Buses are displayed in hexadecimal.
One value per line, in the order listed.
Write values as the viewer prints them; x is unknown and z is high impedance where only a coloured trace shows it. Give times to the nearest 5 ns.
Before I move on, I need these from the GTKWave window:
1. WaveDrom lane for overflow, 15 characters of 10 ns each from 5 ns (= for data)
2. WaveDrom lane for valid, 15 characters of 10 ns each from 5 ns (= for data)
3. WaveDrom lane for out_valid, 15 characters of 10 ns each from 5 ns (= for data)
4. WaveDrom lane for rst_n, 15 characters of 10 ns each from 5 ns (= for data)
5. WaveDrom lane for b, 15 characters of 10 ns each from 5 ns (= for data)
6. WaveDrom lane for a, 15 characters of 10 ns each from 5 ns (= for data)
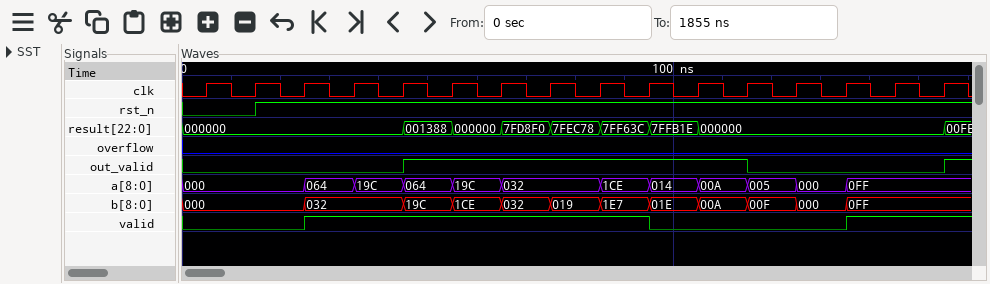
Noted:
{name: 'overflow', wave: '0..............'}
{name: 'valid', wave: '0.1......0...1.'}
{name: 'out_valid', wave: '0...1......0...'}
{name: 'rst_n', wave: '01.............'}
{name: 'b', wave: '=.=.==========.', data: '000 032 19C 1CE 032 019 1E7 01E 00A 00F 000 0FF'}
{name: 'a', wave: '=.=====.======.', data: '000 064 19C 064 19C 032 1CE 014 00A 005 000 0FF'}
